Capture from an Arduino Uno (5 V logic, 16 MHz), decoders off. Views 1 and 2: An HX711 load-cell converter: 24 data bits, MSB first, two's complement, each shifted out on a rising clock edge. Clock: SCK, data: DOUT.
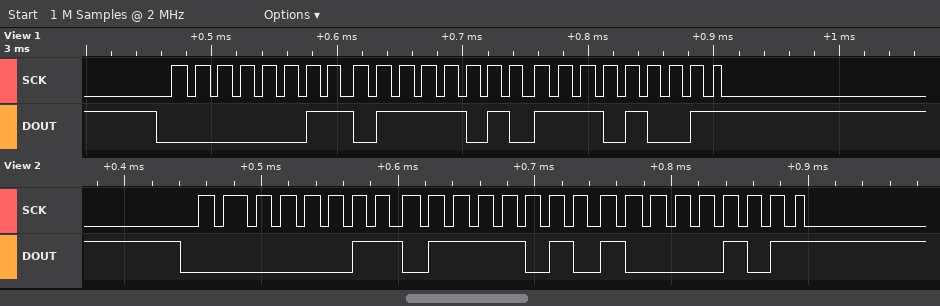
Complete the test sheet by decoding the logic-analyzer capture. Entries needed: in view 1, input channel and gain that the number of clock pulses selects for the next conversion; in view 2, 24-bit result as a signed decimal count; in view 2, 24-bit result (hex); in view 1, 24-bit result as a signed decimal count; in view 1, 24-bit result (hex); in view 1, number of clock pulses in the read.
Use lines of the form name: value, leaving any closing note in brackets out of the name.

in view 1, input channel and gain that the number of clock pulses selects for the next conversion: channel A, gain 128
in view 2, 24-bit result as a signed decimal count: 227973
in view 2, 24-bit result: 0x037A85
in view 1, 24-bit result as a signed decimal count: 228073
in view 1, 24-bit result: 0x037AE9
in view 1, number of clock pulses in the read: 25
